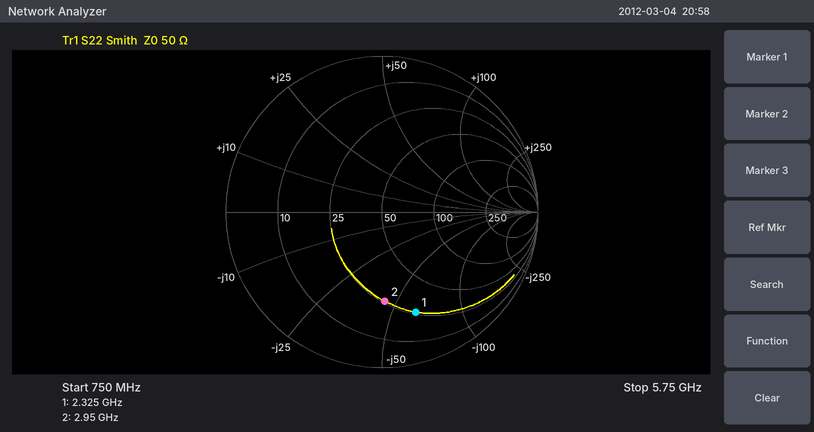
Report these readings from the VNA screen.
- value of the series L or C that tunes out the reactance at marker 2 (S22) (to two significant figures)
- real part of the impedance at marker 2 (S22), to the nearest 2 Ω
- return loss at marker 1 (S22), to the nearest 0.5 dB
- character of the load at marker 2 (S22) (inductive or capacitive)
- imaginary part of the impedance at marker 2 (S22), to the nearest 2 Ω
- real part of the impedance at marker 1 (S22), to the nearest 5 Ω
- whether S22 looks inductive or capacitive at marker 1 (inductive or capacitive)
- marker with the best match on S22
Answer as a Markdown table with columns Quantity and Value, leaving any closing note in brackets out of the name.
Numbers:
| Quantity | Value |
|---|---|
| value of the series L or C that tunes out the reactance at marker 2 (S22) | 2.4 nH |
| real part of the impedance at marker 2 (S22), to the nearest 2 Ω | 26 Ω |
| return loss at marker 1 (S22), to the nearest 0.5 dB | 3.5 dB |
| character of the load at marker 2 (S22) | capacitive |
| imaginary part of the impedance at marker 2 (S22), to the nearest 2 Ω | -44 Ω |
| real part of the impedance at marker 1 (S22), to the nearest 5 Ω | 25 Ω |
| whether S22 looks inductive or capacitive at marker 1 | capacitive |
| marker with the best match on S22 | marker 2 |
